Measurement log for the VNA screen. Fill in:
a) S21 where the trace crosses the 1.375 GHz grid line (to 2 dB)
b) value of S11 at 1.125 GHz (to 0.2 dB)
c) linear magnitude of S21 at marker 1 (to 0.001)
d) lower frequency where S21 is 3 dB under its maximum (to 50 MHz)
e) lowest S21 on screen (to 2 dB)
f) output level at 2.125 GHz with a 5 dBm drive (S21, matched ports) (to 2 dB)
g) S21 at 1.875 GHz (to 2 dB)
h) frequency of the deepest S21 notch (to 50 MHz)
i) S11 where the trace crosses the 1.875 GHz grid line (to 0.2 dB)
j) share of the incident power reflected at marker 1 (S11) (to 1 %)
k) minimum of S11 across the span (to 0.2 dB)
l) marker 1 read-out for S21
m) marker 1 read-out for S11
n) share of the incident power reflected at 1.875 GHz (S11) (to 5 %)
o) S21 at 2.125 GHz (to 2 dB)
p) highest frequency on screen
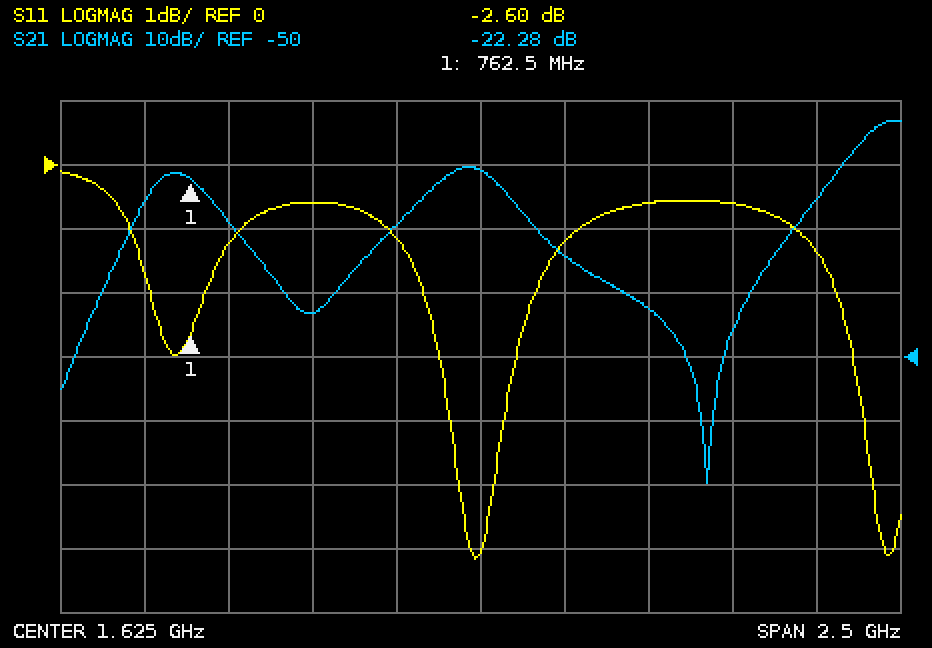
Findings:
-30 dB
-0.6 dB
0.077
2.75 GHz
-70 dB
-38 dBm
-34 dB
2.30 GHz
-1.2 dB
55 %
-6.2 dB
-22.28 dB
-2.60 dB
75 %
-42 dB
2.875 GHz
